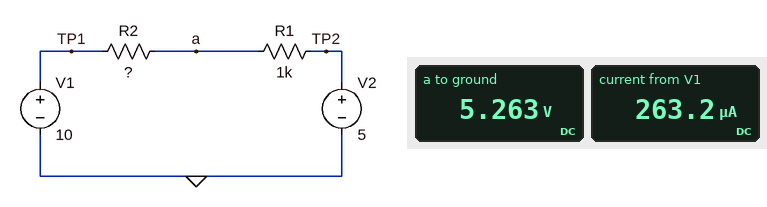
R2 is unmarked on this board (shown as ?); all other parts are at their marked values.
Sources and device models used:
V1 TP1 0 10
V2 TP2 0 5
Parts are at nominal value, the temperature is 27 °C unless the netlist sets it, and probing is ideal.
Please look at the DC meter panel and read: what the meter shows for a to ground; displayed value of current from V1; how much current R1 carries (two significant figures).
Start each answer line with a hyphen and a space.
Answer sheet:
- 5.263 V
- 263.2 µA
- 260 µA
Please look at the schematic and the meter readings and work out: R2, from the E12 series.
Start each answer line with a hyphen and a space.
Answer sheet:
- 18 kΩ
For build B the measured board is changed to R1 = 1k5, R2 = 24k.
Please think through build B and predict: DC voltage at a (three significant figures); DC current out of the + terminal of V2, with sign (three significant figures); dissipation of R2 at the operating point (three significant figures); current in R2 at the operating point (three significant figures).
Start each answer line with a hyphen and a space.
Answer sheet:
- 5.29 V
- -196 µA
- 923 µW
- 196 µA
